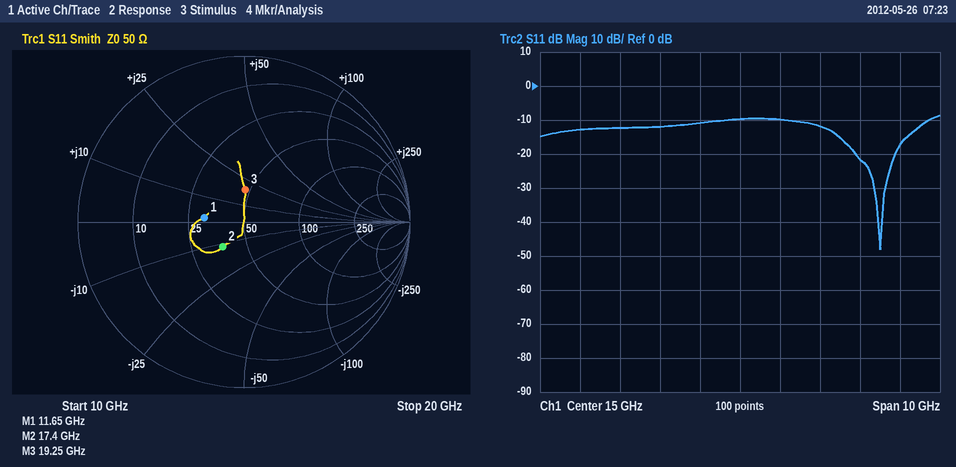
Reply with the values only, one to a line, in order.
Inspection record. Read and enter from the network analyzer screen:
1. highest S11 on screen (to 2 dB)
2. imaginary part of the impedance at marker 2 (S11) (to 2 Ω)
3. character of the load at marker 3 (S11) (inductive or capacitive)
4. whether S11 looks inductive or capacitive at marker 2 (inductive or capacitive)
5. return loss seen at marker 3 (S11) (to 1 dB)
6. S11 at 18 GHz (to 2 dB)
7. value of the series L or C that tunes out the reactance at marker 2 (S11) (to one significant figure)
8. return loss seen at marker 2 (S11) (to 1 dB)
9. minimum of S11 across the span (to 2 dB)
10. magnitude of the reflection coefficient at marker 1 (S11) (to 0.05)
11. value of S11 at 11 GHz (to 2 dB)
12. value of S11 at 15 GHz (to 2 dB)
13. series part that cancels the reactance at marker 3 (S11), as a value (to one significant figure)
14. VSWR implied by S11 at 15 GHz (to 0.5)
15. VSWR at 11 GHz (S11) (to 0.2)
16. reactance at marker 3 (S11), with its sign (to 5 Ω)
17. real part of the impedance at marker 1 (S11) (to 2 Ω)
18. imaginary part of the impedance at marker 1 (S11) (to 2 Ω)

-8 dB
-12 Ω
inductive
capacitive
14 dB
-22 dB
100 pH
14 dB
-48 dB
0.25
-12 dB
-10 dB
400 fF
2.0
1.6
+20 Ω
30 Ω
+2 Ω
